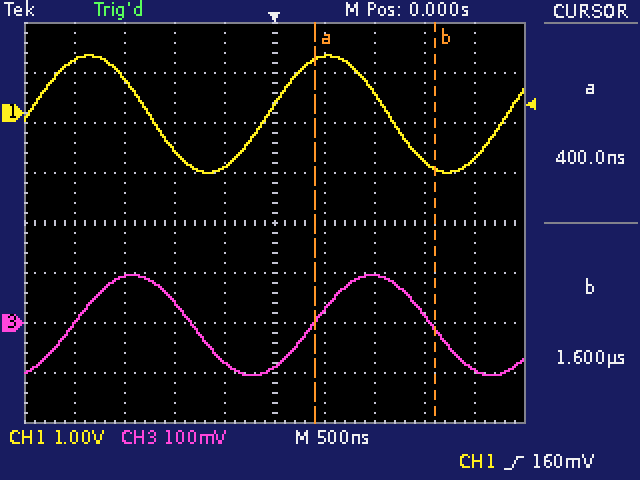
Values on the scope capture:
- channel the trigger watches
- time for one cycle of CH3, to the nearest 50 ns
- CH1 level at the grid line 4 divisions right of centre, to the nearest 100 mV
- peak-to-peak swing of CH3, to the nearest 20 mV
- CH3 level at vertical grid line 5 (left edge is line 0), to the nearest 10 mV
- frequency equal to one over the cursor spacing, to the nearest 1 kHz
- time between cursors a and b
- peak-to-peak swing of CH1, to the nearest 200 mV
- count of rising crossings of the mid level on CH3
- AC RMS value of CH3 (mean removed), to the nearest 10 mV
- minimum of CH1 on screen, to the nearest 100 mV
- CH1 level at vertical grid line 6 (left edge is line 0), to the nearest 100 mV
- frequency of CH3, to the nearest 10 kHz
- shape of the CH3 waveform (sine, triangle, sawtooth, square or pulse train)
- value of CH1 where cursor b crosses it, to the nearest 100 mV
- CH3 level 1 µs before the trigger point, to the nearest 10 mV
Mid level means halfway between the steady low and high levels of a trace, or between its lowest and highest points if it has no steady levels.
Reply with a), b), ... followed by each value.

a) CH1
b) 2.40 µs
c) -900 mV
d) 200 mV
e) -90 mV
f) 833 kHz
g) 1.20 µs
h) 2.4 V
i) 2
j) 70 mV
k) -1.2 V
l) 1.1 V
m) 420 kHz
n) sine
o) -1.1 V
p) 40 mV
